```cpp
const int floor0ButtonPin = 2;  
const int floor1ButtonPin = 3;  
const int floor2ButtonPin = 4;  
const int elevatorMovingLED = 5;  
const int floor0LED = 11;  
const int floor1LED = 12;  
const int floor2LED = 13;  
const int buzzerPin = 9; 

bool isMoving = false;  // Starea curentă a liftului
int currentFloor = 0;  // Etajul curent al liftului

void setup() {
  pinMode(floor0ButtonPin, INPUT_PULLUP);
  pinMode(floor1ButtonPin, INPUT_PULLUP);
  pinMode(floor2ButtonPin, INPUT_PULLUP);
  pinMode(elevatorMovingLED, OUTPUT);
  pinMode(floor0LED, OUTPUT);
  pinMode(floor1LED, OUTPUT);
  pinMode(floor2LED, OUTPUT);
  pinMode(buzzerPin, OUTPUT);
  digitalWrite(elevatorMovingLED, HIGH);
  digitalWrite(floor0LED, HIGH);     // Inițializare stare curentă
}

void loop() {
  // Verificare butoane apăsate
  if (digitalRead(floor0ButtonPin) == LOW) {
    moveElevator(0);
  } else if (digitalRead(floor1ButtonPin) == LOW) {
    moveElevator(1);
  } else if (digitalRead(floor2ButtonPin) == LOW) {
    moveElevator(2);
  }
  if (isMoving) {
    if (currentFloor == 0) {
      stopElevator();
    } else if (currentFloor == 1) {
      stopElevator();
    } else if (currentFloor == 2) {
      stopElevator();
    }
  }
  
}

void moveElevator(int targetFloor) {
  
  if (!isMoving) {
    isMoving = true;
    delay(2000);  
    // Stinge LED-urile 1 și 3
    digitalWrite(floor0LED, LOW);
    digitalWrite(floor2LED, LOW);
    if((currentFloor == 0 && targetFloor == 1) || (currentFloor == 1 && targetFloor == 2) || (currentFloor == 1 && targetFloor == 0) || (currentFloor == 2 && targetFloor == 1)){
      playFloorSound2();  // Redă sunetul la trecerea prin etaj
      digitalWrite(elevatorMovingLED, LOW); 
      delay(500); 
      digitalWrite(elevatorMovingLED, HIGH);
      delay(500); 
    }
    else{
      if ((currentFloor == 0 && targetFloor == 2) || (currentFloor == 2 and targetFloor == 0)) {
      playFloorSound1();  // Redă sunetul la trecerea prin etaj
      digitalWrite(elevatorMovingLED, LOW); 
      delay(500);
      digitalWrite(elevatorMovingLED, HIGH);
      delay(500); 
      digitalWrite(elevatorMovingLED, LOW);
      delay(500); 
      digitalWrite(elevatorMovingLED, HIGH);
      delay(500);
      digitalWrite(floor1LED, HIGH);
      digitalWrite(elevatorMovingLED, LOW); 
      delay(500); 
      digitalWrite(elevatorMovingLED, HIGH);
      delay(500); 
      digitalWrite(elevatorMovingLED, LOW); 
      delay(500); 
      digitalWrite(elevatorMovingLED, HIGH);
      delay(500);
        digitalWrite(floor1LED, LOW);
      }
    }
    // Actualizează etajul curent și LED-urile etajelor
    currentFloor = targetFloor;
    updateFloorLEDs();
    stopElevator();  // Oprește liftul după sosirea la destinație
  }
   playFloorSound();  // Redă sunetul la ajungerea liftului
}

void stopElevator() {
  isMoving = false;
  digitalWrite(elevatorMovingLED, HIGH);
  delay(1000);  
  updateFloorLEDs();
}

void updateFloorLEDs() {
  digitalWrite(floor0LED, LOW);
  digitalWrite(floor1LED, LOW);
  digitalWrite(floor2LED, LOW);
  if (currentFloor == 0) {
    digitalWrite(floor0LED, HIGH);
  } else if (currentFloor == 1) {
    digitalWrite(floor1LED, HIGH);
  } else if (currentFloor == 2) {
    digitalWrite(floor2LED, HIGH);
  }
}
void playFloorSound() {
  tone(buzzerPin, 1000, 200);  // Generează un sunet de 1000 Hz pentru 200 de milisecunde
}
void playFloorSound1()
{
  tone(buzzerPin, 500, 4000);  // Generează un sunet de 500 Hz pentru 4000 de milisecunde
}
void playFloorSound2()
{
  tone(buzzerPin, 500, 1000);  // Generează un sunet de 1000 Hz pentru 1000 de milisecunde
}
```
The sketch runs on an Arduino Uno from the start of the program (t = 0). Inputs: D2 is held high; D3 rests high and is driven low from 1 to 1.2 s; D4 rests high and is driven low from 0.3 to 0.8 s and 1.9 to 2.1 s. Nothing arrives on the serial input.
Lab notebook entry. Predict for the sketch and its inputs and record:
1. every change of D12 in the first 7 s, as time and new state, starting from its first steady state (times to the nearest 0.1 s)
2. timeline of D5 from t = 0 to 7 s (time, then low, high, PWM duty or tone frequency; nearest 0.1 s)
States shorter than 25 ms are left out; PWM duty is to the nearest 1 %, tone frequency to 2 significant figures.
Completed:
0 s low; 4.3 s high; 6.3 s low
0 s high; 2.3 s low; 2.8 s high; 3.3 s low; 3.8 s high; 4.3 s low; 4.8 s high; 5.3 s low; 5.8 s high
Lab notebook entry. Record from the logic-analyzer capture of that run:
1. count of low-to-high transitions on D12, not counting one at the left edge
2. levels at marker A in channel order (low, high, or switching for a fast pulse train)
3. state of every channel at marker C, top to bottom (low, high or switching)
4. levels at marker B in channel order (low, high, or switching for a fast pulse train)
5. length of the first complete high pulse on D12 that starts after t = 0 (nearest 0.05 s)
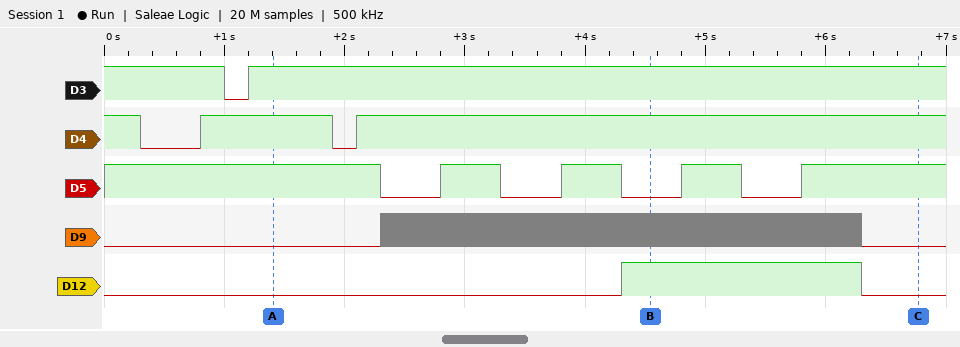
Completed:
1
D3 high, D4 high, D5 high, D9 low, D12 low
D3 high, D4 high, D5 high, D9 low, D12 low
D3 high, D4 high, D5 low, D9 switching, D12 high
2.00 s
